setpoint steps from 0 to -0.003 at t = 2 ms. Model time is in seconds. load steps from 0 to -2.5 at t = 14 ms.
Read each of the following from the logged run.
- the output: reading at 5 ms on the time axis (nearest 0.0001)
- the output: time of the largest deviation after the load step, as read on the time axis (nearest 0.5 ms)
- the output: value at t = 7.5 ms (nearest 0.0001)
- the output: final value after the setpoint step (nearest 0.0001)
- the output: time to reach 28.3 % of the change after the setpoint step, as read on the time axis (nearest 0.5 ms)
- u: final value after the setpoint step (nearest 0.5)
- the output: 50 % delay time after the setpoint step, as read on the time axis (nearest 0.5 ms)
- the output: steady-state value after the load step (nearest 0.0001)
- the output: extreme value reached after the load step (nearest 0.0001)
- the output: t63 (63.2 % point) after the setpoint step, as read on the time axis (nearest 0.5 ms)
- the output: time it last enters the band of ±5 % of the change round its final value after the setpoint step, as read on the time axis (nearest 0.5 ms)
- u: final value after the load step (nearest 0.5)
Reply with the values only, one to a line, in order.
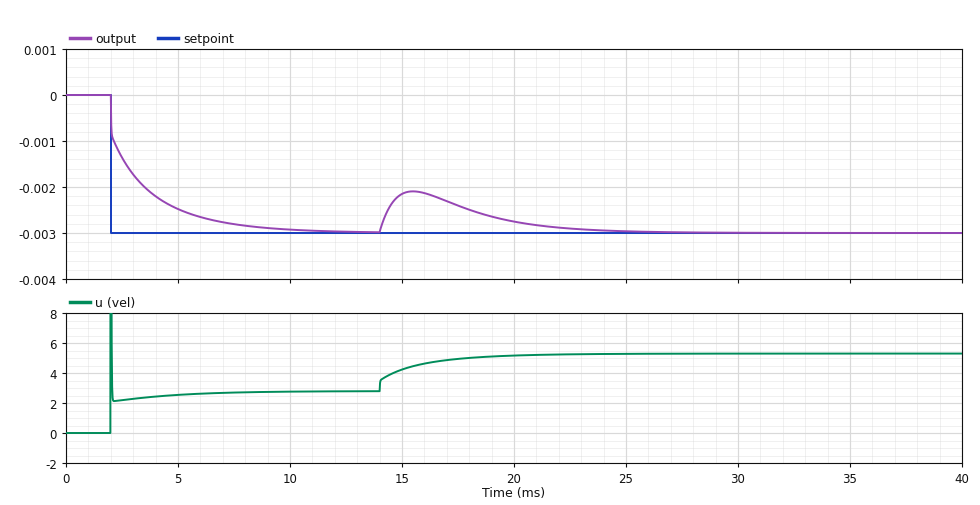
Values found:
-0.0025
15.5 ms
-0.0028
-0.0030
2.0 ms
3.0
2.5 ms
-0.0030
-0.0021
3.5 ms
8.0 ms
5.5
